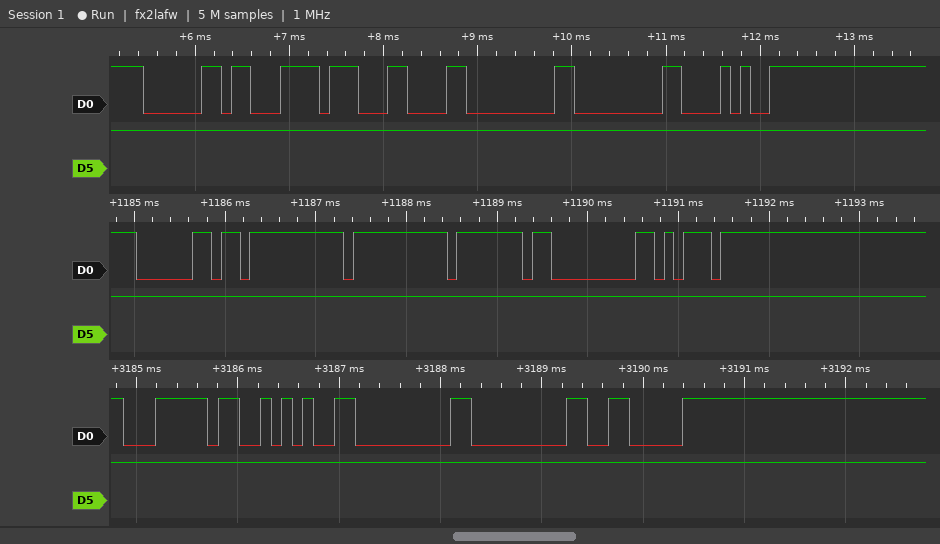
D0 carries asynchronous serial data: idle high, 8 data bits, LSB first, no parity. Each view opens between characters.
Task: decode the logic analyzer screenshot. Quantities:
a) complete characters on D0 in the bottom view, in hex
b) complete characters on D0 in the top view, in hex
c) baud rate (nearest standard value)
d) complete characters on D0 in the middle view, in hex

7C, 2A, 00, 00, 06
60, BC, 0C, 00, 00, 28
9600 baud
60, FF, FF, 7F, 00, DD
